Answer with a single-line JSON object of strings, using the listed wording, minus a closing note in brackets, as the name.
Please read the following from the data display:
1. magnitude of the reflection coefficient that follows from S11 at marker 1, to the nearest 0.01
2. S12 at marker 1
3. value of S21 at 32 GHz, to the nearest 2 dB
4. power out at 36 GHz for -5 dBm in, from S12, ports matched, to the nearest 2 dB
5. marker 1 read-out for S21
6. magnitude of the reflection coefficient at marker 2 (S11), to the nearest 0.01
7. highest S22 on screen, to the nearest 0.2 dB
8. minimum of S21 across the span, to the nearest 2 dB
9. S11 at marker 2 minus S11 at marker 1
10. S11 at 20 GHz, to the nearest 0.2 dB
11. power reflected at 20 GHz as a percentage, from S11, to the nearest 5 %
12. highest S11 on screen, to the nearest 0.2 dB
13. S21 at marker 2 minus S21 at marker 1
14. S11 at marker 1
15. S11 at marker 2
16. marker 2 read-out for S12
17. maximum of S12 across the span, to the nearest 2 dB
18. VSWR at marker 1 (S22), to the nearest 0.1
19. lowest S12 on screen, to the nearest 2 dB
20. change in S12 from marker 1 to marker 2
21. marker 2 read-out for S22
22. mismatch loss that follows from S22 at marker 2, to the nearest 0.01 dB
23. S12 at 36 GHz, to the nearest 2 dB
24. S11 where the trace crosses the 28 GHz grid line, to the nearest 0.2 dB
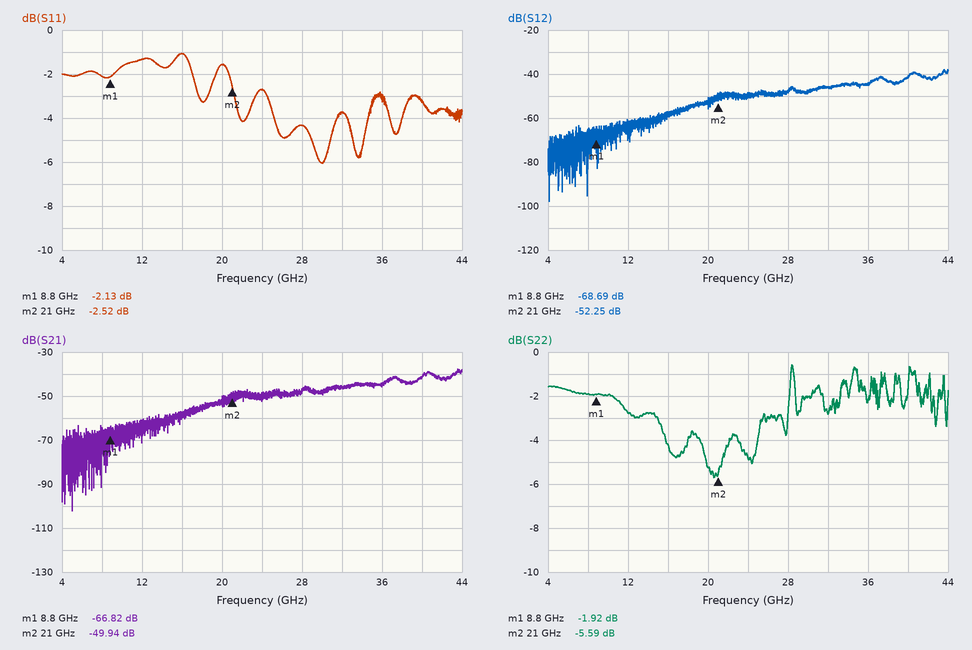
{"magnitude of the reflection coefficient that follows from S11 at marker 1, to the nearest 0.01": "0.78", "S12 at marker 1": "-68.69 dB", "value of S21 at 32 GHz, to the nearest 2 dB": "-46 dB", "power out at 36 GHz for -5 dBm in, from S12, ports matched, to the nearest 2 dB": "-50 dBm", "marker 1 read-out for S21": "-66.82 dB", "magnitude of the reflection coefficient at marker 2 (S11), to the nearest 0.01": "0.75", "highest S22 on screen, to the nearest 0.2 dB": "-0.6 dB", "minimum of S21 across the span, to the nearest 2 dB": "-102 dB", "S11 at marker 2 minus S11 at marker 1": "-0.39 dB", "S11 at 20 GHz, to the nearest 0.2 dB": "-1.6 dB", "power reflected at 20 GHz as a percentage, from S11, to the nearest 5 %": "70 %", "highest S11 on screen, to the nearest 0.2 dB": "-1.0 dB", "S21 at marker 2 minus S21 at marker 1": "16.88 dB", "S11 at marker 1": "-2.13 dB", "S11 at marker 2": "-2.52 dB", "marker 2 read-out for S12": "-52.25 dB", "maximum of S12 across the span, to the nearest 2 dB": "-38 dB", "VSWR at marker 1 (S22), to the nearest 0.1": "9.1", "lowest S12 on screen, to the nearest 2 dB": "-98 dB", "change in S12 from marker 1 to marker 2": "16.44 dB", "marker 2 read-out for S22": "-5.59 dB", "mismatch loss that follows from S22 at marker 2, to the nearest 0.01 dB": "1.40 dB", "S12 at 36 GHz, to the nearest 2 dB": "-44 dB", "S11 where the trace crosses the 28 GHz grid line, to the nearest 0.2 dB": "-4.4 dB"}
